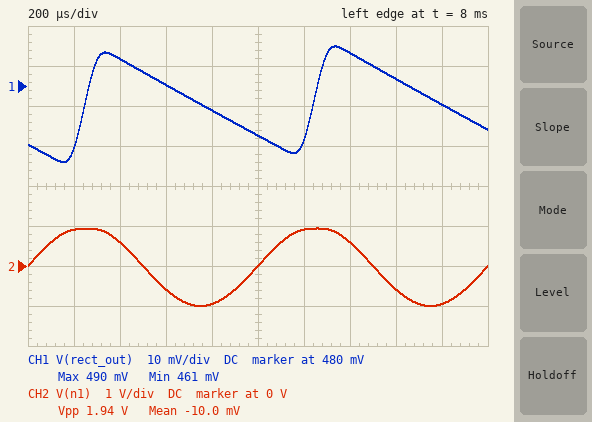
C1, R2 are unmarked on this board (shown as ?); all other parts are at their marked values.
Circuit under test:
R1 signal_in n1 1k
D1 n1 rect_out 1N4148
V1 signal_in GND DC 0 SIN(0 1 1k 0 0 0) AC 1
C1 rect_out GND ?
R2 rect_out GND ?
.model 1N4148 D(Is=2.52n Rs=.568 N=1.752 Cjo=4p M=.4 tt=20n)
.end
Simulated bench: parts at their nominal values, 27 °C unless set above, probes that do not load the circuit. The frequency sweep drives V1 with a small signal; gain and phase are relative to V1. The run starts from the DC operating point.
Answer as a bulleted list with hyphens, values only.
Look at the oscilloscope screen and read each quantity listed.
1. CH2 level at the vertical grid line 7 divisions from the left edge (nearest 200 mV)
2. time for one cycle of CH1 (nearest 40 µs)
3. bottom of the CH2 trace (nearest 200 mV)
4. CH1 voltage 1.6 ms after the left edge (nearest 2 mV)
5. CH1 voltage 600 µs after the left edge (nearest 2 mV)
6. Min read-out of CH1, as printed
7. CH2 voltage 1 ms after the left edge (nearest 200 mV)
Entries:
- 600 mV
- 1.00 ms
- -1.0 V
- 482 mV
- 480 mV
- 461 mV
- 0 V
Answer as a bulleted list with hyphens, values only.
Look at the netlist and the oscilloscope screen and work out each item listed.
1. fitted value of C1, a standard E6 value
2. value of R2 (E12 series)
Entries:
- 220 nF
- 68 kΩ
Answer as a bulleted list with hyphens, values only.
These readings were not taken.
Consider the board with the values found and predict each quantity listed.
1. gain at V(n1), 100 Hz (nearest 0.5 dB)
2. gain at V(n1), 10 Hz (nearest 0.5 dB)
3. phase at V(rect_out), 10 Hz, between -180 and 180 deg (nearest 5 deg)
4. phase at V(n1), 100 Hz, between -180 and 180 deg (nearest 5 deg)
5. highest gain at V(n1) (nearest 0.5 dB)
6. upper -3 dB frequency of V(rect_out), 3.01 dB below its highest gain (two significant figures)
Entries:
- 0 dB
- 0 dB
- -45 deg
- 0 deg
- 0 dB
- 11 Hz
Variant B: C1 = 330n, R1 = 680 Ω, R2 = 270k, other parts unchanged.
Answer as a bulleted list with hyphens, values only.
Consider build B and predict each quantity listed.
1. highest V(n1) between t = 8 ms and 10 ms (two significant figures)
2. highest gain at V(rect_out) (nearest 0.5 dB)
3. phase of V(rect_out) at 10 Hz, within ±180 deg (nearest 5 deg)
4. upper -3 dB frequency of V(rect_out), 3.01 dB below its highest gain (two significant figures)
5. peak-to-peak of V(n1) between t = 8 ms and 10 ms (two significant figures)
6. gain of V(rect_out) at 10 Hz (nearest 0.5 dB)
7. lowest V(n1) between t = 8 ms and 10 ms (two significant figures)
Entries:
- 970 mV
- -36.5 dB
- -80 deg
- 1.8 Hz
- 2.0 V
- -51.5 dB
- -1.0 V
